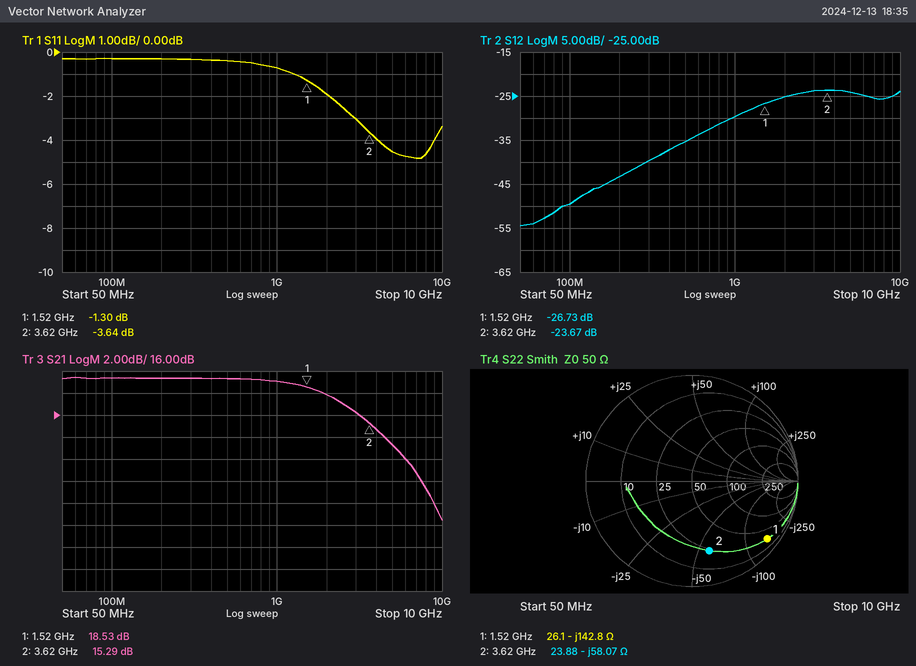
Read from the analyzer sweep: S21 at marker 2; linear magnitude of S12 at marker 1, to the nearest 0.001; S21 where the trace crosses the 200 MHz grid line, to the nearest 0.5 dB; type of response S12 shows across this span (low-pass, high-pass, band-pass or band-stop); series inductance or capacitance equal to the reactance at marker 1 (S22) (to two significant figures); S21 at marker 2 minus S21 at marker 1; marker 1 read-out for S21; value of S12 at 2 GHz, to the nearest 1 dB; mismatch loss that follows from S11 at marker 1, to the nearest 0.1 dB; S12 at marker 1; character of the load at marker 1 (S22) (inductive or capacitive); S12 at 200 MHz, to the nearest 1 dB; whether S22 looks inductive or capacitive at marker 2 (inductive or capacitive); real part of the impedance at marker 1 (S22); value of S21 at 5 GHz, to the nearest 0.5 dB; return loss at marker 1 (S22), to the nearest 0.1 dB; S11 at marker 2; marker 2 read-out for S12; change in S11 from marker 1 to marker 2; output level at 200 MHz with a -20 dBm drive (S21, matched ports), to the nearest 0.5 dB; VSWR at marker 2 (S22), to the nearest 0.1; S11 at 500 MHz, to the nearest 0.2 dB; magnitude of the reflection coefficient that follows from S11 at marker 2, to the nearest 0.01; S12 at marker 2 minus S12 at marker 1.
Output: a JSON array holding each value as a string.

["15.29 dB", "0.046", "19.5 dB", "high-pass", "730 fF", "-3.24 dB", "18.53 dB", "-25 dB", "5.9 dB", "-26.73 dB", "capacitive", "-43 dB", "capacitive", "26.1 Ω", "13.5 dB", "1.0 dB", "-3.64 dB", "-23.67 dB", "-2.34 dB", "-0.5 dBm", "5.2", "-0.4 dB", "0.66", "3.06 dB"]
